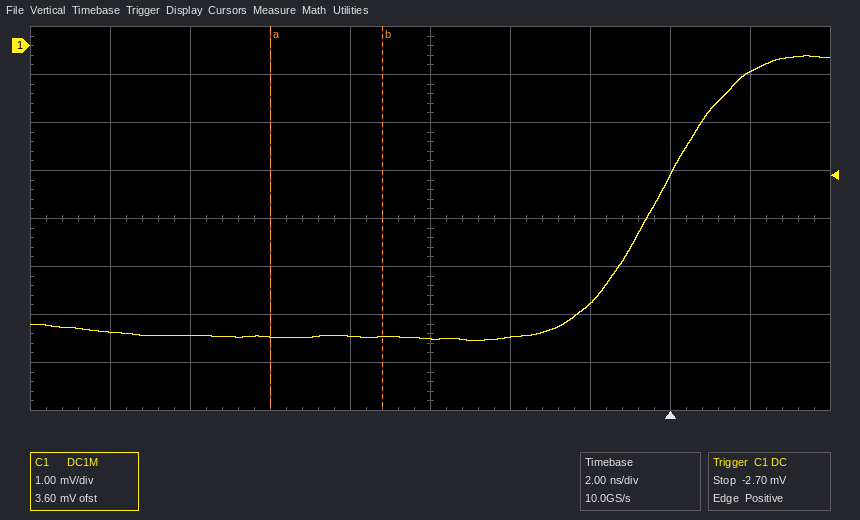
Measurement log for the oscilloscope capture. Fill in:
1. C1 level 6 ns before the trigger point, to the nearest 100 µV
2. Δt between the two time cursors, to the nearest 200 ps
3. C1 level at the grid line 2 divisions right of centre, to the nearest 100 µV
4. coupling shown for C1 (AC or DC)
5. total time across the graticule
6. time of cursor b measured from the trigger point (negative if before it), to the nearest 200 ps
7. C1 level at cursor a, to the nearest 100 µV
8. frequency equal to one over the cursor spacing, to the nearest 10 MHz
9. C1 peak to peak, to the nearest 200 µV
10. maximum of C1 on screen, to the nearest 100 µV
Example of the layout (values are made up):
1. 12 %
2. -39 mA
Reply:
1. -6.1 mV
2. 2.8 ns
3. -5.4 mV
4. DC
5. 20 ns
6. -7.2 ns
7. -6.1 mV
8. 360 MHz
9. 6.0 mV
10. -200 µV
